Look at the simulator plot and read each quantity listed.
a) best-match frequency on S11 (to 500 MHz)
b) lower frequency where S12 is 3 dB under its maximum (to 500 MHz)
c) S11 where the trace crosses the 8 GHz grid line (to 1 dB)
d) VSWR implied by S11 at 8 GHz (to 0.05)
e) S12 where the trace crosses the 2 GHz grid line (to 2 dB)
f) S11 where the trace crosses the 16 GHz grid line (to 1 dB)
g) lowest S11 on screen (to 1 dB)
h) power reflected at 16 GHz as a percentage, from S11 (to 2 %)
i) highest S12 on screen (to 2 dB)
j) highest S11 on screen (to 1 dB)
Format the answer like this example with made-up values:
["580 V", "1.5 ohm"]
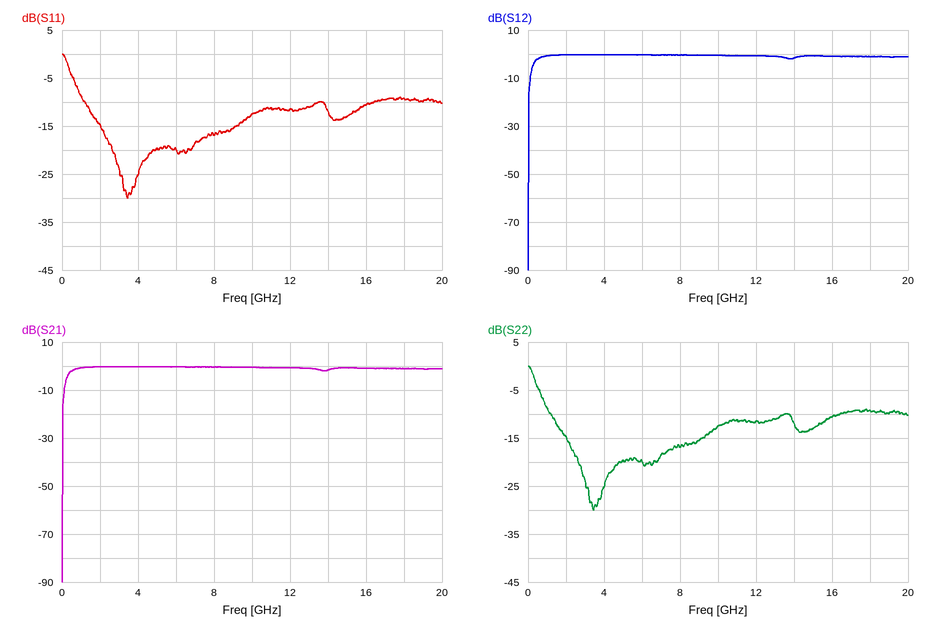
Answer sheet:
["3.5 GHz", "500 MHz", "-17 dB", "1.35", "0 dB", "-11 dB", "-30 dB", "8 %", "0 dB", "0 dB"]
